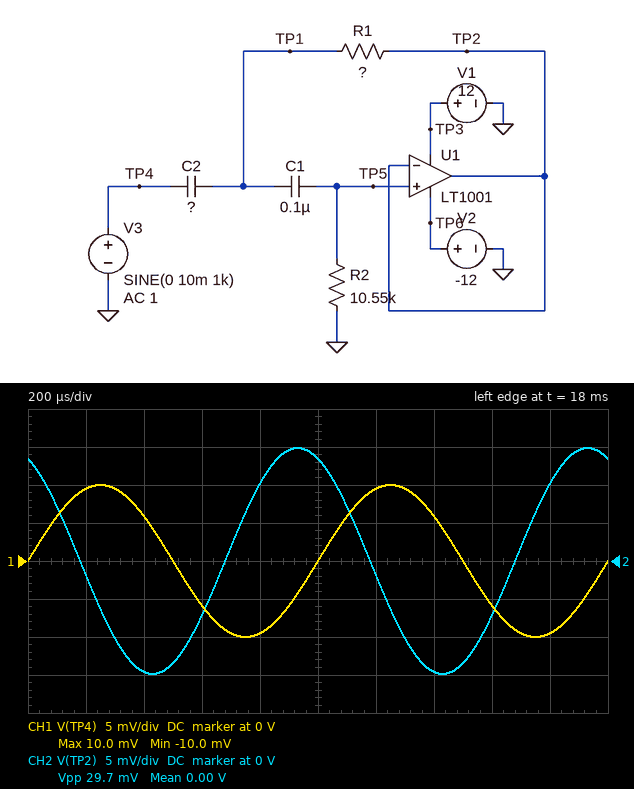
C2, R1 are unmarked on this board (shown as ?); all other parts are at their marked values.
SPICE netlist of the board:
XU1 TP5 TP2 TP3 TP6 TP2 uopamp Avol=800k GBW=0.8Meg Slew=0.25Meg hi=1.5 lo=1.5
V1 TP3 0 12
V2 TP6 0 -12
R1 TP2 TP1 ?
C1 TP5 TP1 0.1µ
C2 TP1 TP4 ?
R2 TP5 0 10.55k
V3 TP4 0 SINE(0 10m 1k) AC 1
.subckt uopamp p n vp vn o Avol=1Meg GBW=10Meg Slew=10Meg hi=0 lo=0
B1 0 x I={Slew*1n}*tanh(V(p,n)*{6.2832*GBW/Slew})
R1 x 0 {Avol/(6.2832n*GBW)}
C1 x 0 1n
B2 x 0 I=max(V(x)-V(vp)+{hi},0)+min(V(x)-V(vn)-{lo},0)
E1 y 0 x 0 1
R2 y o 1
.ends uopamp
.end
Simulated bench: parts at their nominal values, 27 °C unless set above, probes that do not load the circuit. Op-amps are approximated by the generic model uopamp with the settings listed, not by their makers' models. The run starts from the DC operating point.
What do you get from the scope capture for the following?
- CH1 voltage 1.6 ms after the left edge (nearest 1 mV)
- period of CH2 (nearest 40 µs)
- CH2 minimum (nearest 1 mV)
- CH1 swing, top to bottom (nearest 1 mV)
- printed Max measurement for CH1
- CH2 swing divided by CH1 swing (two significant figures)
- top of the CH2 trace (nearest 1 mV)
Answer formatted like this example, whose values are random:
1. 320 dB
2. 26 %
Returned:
1. -6 mV
2. 1.00 ms
3. -15 mV
4. 20 mV
5. 10.0 mV
6. 1.5
7. 15 mV
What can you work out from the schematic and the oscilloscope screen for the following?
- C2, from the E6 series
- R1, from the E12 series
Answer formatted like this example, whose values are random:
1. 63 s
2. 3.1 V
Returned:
1. 33 nF
2. 560 Ω
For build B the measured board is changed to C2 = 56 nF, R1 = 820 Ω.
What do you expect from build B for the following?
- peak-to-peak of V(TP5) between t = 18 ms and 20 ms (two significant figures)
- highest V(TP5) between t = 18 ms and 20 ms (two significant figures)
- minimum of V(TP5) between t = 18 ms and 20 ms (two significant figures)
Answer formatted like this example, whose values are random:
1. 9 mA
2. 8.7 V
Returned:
1. 31 mV
2. 16 mV
3. -16 mV
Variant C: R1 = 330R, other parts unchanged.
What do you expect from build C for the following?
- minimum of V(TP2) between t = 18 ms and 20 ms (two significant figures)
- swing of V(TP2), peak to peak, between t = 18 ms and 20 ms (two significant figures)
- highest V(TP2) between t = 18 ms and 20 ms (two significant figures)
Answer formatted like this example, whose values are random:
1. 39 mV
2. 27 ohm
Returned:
1. -7.5 mV
2. 15 mV
3. 7.5 mV
